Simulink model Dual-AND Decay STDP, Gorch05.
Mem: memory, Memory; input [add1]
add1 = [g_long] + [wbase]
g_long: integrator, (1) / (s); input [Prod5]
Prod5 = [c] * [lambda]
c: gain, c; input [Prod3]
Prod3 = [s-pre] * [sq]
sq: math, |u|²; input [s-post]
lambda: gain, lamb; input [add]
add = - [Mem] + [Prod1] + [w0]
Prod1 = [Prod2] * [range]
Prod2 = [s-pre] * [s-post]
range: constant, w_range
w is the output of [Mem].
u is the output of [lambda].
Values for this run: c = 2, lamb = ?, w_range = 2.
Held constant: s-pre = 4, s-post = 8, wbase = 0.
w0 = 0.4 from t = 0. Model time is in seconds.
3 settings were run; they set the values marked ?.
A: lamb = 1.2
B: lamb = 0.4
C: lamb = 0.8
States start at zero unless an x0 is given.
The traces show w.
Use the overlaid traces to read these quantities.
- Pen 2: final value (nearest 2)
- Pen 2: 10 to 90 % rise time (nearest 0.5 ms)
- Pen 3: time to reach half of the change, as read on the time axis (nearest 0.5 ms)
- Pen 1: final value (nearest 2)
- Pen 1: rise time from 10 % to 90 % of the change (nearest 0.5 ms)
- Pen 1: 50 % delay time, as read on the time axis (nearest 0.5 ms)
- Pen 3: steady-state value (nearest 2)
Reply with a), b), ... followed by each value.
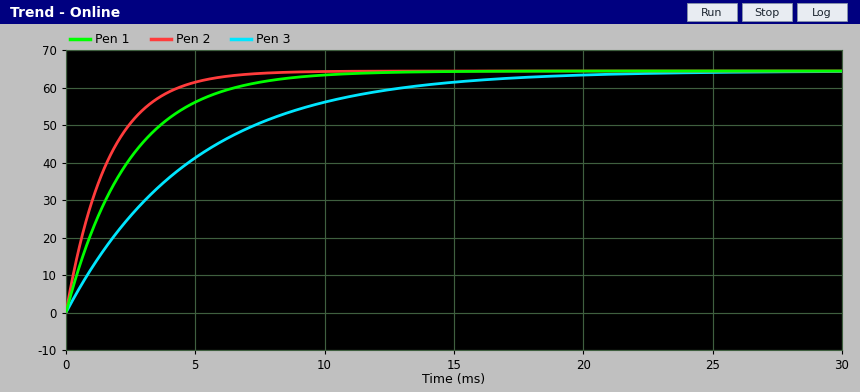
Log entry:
a) 64
b) 3.5 ms
c) 3.5 ms
d) 64
e) 5.5 ms
f) 1.5 ms
g) 64
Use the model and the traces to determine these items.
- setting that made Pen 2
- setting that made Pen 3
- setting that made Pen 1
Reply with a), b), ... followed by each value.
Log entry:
a) A
b) B
c) C
